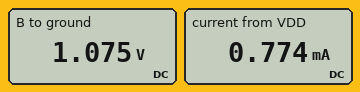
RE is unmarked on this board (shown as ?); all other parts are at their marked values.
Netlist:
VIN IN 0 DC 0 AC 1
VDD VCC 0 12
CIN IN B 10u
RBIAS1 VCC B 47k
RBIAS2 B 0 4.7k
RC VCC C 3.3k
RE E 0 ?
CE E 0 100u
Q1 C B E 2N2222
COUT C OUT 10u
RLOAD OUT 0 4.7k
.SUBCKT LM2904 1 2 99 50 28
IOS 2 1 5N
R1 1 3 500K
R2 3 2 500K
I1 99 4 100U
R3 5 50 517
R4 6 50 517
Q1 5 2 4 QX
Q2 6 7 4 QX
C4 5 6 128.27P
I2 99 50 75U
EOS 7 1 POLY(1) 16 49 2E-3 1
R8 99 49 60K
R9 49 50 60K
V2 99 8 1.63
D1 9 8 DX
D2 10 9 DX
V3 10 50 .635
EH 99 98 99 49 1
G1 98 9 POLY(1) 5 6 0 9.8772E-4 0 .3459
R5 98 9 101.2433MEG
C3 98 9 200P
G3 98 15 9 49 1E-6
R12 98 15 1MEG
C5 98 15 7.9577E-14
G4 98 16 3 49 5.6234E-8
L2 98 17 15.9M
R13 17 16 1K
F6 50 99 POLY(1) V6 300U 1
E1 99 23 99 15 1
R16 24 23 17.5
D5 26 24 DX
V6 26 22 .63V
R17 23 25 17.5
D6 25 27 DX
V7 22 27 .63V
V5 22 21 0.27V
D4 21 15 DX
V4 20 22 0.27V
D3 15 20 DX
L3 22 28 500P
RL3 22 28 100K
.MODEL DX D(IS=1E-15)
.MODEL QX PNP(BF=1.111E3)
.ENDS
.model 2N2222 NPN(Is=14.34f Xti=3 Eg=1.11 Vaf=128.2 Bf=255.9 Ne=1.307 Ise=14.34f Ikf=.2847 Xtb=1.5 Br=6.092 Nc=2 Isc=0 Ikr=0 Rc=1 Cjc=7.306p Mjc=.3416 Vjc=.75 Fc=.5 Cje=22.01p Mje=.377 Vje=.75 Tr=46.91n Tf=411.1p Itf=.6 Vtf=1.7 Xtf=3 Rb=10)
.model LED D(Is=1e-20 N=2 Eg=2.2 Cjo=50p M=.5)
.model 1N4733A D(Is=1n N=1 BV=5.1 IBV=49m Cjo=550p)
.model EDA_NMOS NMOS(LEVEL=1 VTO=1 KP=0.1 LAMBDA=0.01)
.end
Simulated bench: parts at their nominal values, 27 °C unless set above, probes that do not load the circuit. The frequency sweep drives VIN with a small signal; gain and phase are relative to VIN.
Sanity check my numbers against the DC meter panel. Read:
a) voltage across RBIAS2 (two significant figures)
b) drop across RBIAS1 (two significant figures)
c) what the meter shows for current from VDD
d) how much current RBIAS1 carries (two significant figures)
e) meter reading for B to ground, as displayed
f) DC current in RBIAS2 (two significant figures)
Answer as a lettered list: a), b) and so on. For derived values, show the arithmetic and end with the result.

a) 1.075 V = 1.1 V
b) 12 V - 1.075 V = 11 V
c) 0.774 mA
d) (12 V - 1.075 V) / 47 kΩ = 230 µA
e) 1.075 V
f) (1.075 V) / 4.7 kΩ = 230 µA
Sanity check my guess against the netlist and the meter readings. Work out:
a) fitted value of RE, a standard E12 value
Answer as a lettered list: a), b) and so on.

a) 820 Ω
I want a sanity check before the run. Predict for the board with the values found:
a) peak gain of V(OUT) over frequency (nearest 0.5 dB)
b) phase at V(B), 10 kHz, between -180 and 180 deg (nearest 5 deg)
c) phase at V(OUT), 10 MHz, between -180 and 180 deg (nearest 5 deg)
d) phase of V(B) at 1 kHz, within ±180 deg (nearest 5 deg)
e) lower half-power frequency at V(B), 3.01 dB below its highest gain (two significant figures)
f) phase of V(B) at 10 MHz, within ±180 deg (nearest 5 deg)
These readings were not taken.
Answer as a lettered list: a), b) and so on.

a) 32.0 dB
b) 0 deg
c) 155 deg
d) 0 deg
e) 4.1 Hz
f) 0 deg
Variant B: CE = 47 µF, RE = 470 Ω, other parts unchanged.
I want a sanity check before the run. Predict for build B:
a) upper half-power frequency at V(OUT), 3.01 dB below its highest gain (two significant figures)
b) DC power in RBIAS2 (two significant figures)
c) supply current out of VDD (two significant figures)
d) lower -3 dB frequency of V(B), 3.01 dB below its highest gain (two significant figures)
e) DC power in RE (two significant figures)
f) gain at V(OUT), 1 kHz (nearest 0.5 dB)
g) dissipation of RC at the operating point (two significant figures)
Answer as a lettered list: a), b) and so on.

a) 19 MHz
b) 240 µW
c) 1.1 mA
d) 4.0 Hz
e) 380 µW
f) 36.5 dB
g) 2.7 mW
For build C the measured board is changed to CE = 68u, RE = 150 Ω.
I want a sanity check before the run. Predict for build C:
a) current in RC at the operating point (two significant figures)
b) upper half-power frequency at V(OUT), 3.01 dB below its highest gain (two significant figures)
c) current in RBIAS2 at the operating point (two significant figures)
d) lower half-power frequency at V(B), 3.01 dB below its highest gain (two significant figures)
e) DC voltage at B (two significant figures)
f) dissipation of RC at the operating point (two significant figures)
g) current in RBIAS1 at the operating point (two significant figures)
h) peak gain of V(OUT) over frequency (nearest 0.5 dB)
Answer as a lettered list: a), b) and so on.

a) 2.4 mA
b) 10 MHz
c) 220 µA
d) 4.5 Hz
e) 1.0 V
f) 19 mW
g) 230 µA
h) 44.5 dB
